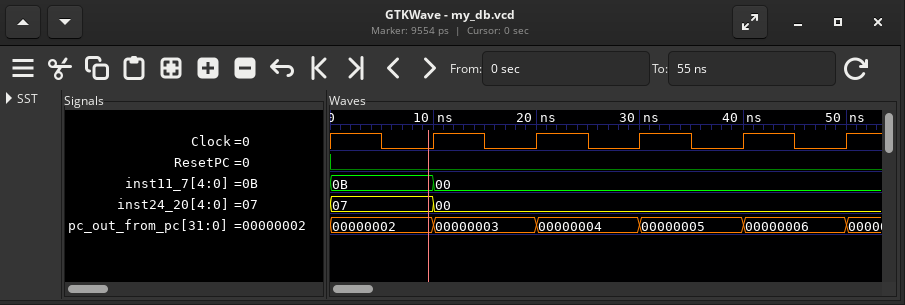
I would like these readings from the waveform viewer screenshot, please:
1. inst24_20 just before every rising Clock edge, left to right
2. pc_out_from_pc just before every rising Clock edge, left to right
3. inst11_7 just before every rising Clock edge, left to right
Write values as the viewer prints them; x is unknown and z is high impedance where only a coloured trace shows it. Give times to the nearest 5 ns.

07, 00, 00, 00, 00
00000002, 00000003, 00000004, 00000005, 00000006
0B, 00, 00, 00, 00
